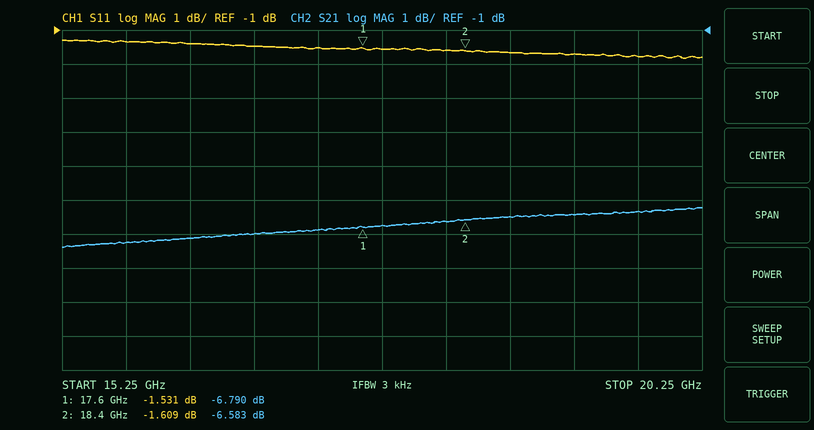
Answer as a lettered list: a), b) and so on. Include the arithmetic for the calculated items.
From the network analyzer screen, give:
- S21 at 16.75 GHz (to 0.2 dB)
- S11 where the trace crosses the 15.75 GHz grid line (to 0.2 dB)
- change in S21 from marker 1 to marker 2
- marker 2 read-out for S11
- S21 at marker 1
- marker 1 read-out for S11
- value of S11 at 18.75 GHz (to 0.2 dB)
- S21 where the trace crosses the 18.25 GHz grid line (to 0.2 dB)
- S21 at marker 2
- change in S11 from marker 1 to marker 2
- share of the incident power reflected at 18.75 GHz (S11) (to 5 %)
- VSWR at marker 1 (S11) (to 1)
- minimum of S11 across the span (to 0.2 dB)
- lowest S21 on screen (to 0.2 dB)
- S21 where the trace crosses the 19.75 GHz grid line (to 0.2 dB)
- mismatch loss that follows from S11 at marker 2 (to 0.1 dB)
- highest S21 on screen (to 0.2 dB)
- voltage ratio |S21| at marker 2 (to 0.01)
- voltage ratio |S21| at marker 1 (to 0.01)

a) -7.0 dB
b) -1.4 dB
c) -6.583 − (-6.79) = 0.207 dB
d) -1.609 dB
e) -6.790 dB
f) -1.531 dB
g) -1.6 dB
h) -6.6 dB
i) -6.583 dB
j) -1.609 − (-1.531) = -0.078 dB
k) 10^(-1.6/10) ≈ 69.2 %, so 70 % to the nearest 5 %
l) (1 + 0.8384)/(1 − 0.8384) ≈ 11
m) -1.8 dB
n) -7.4 dB
o) -6.4 dB
p) −10 log10(1 − 10^(-1.609/10)) ≈ 5.1 dB
q) -6.2 dB
r) 10^(-6.583/20) ≈ 0.47
s) 10^(-6.79/20) ≈ 0.46
